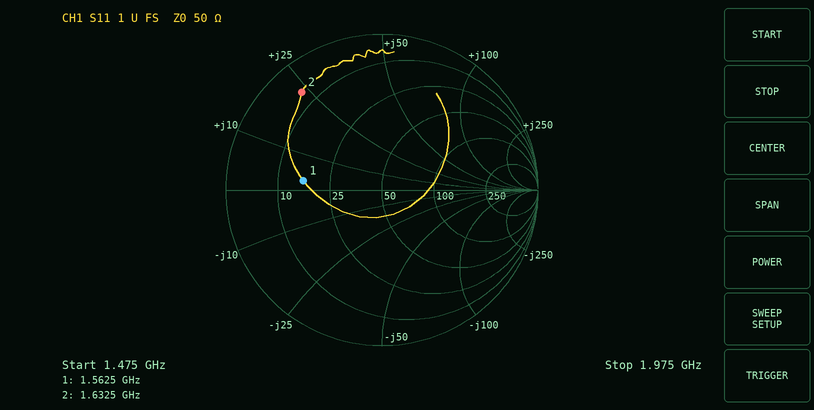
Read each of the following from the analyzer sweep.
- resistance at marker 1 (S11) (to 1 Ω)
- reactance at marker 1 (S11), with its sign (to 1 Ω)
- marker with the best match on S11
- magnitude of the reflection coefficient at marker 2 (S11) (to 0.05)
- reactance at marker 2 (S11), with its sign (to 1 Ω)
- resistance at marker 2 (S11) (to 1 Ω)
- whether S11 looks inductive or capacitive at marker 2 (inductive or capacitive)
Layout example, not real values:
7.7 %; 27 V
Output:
16 Ω; +3 Ω; marker 1; 0.80; +23 Ω; 6 Ω; inductive
